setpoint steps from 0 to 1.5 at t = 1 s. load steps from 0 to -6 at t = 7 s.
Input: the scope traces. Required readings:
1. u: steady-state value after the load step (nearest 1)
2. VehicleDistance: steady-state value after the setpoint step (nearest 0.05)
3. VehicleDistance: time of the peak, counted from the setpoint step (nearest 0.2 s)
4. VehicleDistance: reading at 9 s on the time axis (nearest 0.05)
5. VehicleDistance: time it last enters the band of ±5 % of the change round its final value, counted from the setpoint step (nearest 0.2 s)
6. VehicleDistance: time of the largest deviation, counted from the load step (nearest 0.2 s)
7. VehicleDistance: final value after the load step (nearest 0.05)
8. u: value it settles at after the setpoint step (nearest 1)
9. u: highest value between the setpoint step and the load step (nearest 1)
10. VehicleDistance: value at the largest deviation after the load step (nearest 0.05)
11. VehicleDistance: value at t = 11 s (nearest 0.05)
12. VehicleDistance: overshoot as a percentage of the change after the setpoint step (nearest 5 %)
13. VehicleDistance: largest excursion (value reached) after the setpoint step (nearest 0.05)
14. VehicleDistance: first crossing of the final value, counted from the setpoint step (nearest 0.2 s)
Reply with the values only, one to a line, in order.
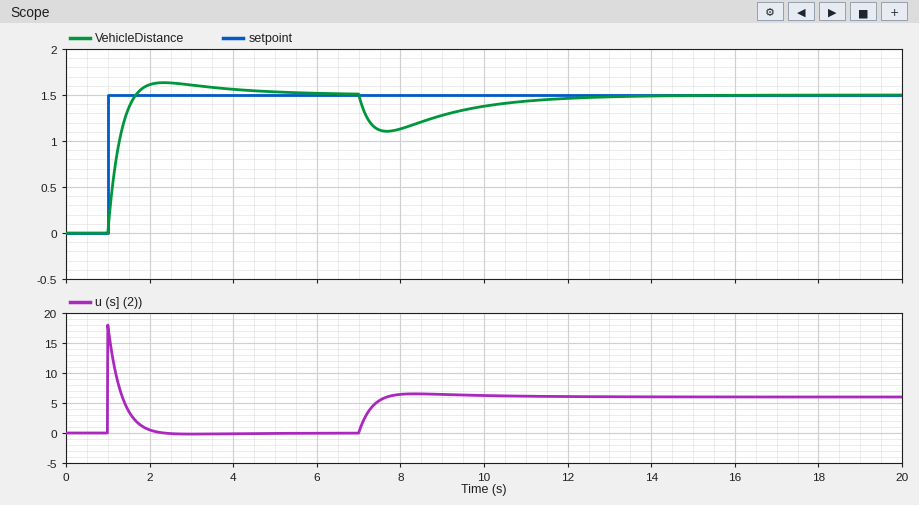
6
1.50
1.4 s
1.30
2.6 s
0.6 s
1.50
0
18
1.10
1.45
10 %
1.65
0.6 s
